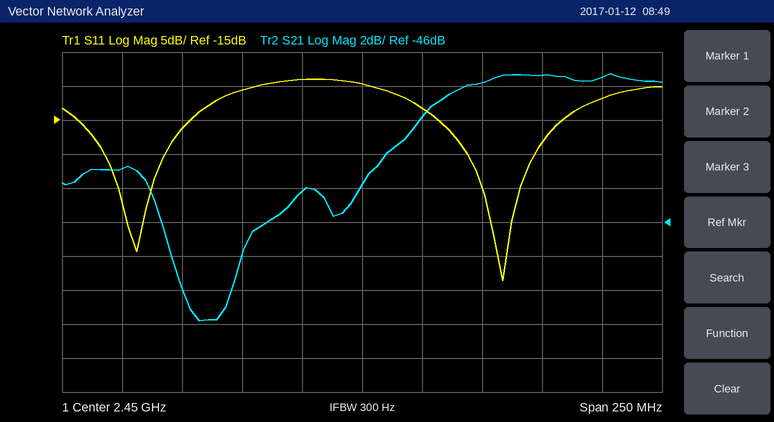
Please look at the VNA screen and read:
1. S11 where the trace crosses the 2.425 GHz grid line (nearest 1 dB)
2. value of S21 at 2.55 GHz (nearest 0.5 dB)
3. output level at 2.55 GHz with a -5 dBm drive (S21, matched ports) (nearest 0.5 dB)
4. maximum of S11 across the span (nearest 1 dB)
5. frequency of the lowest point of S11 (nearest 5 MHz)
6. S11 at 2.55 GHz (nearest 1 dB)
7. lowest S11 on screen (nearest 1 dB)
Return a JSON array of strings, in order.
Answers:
["-9 dB", "-37.5 dB", "-42.5 dBm", "-9 dB", "2.510 GHz", "-12 dB", "-39 dB"]
